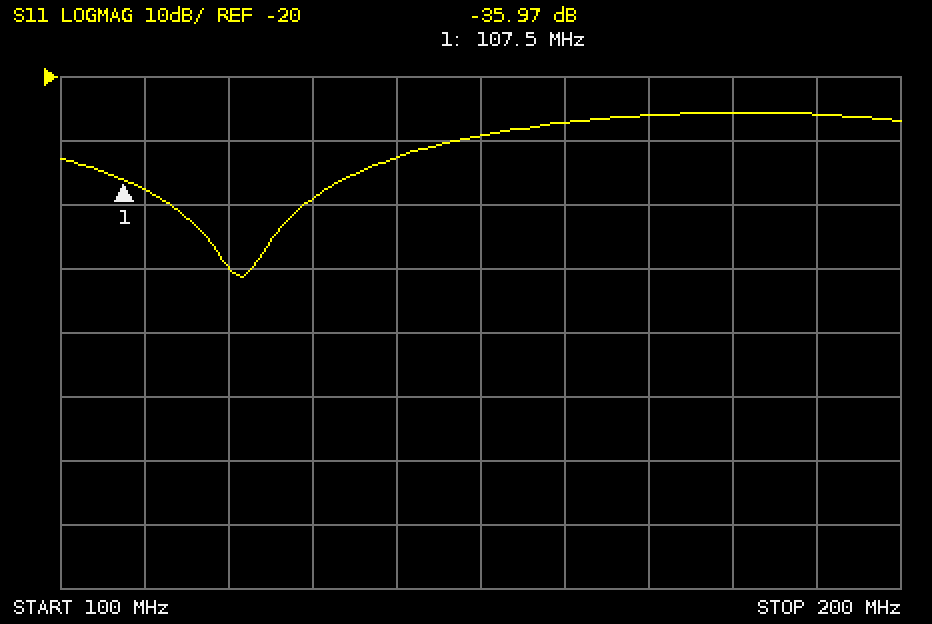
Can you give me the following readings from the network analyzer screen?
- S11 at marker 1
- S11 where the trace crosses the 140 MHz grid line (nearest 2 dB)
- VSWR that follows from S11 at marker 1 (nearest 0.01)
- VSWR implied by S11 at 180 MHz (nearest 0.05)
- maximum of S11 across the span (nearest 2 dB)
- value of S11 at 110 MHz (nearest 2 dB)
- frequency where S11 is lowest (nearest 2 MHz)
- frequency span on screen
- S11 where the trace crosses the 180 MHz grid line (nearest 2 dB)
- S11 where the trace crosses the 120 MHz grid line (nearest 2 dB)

-35.97 dB
-32 dB
1.03
1.10
-26 dB
-38 dB
122 MHz
100 MHz
-26 dB
-50 dB
